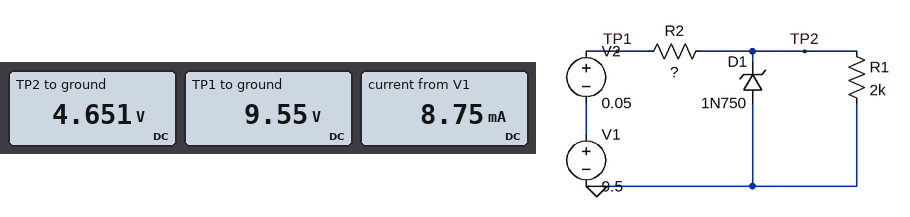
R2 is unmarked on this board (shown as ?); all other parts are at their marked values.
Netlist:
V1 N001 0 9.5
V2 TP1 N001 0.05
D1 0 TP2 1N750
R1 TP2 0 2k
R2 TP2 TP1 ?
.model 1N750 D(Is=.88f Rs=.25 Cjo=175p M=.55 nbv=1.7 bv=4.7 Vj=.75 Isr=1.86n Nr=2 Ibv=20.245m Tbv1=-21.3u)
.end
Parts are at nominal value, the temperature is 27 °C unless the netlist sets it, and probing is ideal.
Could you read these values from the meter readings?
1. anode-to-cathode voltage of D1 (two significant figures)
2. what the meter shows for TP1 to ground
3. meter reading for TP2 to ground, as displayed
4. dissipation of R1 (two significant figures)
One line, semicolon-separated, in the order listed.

-4.7 V; 9.55 V; 4.651 V; 11 mW
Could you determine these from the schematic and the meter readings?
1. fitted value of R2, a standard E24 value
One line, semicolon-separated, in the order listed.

560 Ω
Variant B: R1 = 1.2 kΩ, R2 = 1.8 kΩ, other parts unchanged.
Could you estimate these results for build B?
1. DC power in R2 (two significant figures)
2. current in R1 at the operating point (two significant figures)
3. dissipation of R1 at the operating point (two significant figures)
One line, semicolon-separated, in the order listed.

18 mW; 3.2 mA; 12 mW
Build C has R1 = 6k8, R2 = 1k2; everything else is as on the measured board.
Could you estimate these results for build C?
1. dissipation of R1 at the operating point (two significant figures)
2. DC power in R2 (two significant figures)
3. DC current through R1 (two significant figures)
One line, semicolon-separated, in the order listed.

3.1 mW; 20 mW; 680 µA
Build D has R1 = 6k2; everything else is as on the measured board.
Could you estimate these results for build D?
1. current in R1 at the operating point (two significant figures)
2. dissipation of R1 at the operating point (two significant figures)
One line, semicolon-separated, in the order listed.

750 µA; 3.5 mW
